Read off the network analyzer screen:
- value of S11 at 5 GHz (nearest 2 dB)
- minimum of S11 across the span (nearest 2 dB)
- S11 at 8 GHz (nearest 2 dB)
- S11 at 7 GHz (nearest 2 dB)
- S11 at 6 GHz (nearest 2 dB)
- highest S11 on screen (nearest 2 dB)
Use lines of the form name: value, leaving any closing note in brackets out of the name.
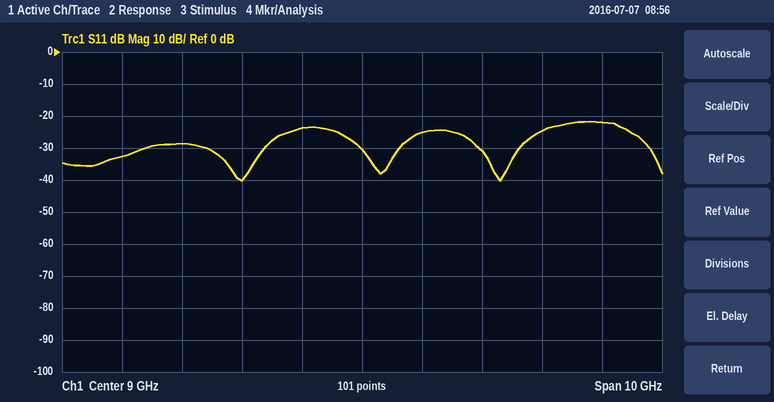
value of S11 at 5 GHz: -32 dB
minimum of S11 across the span: -40 dB
S11 at 8 GHz: -24 dB
S11 at 7 GHz: -40 dB
S11 at 6 GHz: -28 dB
highest S11 on screen: -22 dB
